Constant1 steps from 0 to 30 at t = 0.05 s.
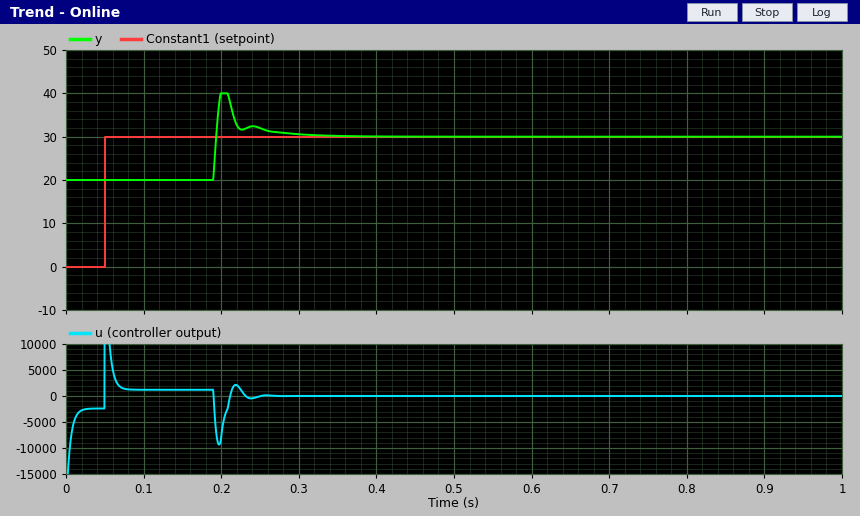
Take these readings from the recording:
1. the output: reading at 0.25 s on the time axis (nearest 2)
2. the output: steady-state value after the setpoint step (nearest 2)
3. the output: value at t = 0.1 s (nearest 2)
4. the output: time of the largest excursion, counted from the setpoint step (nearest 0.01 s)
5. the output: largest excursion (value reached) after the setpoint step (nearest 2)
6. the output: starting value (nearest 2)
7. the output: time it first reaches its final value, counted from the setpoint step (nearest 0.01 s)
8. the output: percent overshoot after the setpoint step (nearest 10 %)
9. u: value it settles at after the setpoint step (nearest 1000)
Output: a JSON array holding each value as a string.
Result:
["32", "30", "20", "0.15 s", "40", "20", "0.14 s", "100 %", "0"]
